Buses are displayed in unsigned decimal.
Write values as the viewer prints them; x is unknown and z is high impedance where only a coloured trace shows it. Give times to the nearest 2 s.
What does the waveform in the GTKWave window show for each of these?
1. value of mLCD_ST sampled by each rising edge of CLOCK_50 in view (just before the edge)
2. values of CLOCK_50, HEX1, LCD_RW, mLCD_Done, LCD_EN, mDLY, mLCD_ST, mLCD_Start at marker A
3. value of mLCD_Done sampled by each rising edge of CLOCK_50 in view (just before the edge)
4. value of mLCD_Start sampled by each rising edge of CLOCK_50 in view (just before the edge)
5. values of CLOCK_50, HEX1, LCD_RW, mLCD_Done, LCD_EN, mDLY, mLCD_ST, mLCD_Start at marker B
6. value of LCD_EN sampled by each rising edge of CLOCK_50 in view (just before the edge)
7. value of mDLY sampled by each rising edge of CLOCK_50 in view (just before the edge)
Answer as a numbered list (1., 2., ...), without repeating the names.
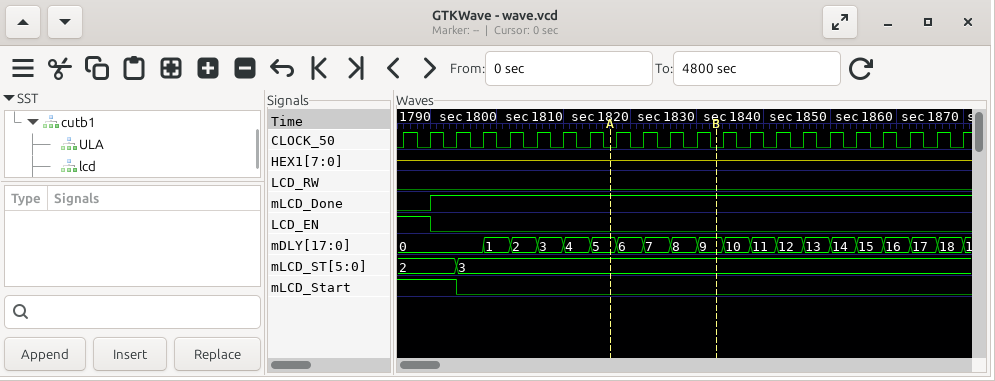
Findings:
1. 2, 2, 2, 3, 3, 3, 3, 3, 3, 3, 3, 3, 3, 3, 3, 3, 3, 3, 3, 3, 3, 3
2. CLOCK_50=0, HEX1=z, LCD_RW=0, mLCD_Done=1, LCD_EN=0, mDLY=5, mLCD_ST=3, mLCD_Start=0
3. 0 0 1 1 1 1 1 1 1 1 1 1 1 1 1 1 1 1 1 1 1 1
4. 1 1 1 0 0 0 0 0 0 0 0 0 0 0 0 0 0 0 0 0 0 0
5. CLOCK_50=0, HEX1=z, LCD_RW=0, mLCD_Done=1, LCD_EN=0, mDLY=9, mLCD_ST=3, mLCD_Start=0
6. 1 1 0 0 0 0 0 0 0 0 0 0 0 0 0 0 0 0 0 0 0 0
7. 0, 0, 0, 0, 1, 2, 3, 4, 5, 6, 7, 8, 9, 10, 11, 12, 13, 14, 15, 16, 17, 18
